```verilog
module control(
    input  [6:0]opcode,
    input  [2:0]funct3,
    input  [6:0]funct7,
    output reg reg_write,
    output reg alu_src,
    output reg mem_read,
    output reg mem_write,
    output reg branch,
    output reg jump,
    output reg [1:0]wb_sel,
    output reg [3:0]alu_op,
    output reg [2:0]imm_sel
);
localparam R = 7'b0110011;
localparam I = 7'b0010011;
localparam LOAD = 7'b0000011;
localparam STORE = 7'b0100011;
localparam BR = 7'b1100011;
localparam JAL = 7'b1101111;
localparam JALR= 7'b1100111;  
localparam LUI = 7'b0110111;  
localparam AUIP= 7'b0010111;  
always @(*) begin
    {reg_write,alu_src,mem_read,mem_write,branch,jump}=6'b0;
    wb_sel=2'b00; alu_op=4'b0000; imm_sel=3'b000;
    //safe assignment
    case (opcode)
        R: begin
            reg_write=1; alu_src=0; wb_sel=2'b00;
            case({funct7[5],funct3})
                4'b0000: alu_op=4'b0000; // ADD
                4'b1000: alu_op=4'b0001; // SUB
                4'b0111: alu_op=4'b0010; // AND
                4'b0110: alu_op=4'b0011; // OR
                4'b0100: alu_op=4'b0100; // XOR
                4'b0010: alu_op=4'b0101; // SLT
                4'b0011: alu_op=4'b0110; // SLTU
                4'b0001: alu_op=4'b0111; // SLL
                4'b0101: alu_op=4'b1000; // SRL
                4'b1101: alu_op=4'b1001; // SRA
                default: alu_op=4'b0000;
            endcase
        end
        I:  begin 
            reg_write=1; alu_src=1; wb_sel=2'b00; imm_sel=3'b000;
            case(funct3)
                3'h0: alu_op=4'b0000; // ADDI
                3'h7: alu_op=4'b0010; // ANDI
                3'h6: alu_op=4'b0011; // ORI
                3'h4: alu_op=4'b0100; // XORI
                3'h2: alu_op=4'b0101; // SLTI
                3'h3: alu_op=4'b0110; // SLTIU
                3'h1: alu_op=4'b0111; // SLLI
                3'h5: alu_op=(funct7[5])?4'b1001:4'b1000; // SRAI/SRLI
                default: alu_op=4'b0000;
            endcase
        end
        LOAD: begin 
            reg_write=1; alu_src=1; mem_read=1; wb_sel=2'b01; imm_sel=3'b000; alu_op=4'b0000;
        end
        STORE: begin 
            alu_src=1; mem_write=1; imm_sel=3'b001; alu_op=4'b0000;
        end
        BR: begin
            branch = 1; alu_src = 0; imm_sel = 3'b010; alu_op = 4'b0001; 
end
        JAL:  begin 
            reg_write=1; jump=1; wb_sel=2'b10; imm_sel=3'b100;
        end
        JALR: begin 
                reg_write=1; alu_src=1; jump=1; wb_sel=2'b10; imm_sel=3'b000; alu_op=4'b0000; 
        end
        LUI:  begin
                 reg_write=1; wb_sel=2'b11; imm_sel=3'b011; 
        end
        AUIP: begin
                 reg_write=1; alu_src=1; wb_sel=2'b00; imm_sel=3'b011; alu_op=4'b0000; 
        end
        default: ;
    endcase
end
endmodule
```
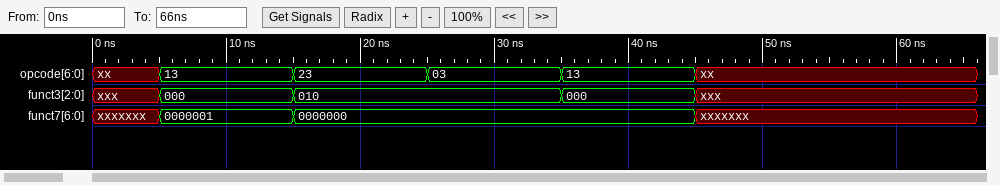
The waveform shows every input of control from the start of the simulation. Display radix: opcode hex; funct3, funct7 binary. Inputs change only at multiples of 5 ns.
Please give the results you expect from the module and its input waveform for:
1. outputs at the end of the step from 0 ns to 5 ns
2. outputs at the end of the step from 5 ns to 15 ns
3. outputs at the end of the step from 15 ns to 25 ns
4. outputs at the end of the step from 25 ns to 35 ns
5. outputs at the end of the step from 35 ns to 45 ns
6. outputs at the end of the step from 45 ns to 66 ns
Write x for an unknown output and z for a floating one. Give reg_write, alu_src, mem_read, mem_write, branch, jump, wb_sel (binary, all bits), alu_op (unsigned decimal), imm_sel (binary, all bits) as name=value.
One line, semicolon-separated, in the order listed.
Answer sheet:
reg_write=x, alu_src=x, mem_read=x, mem_write=x, branch=x, jump=x, wb_sel=x, alu_op=x, imm_sel=x; reg_write=1, alu_src=1, mem_read=0, mem_write=0, branch=0, jump=0, wb_sel=00, alu_op=0, imm_sel=000; reg_write=0, alu_src=1, mem_read=0, mem_write=1, branch=0, jump=0, wb_sel=00, alu_op=0, imm_sel=001; reg_write=1, alu_src=1, mem_read=1, mem_write=0, branch=0, jump=0, wb_sel=01, alu_op=0, imm_sel=000; reg_write=1, alu_src=1, mem_read=0, mem_write=0, branch=0, jump=0, wb_sel=00, alu_op=0, imm_sel=000; reg_write=0, alu_src=0, mem_read=0, mem_write=0, branch=0, jump=0, wb_sel=00, alu_op=0, imm_sel=000
